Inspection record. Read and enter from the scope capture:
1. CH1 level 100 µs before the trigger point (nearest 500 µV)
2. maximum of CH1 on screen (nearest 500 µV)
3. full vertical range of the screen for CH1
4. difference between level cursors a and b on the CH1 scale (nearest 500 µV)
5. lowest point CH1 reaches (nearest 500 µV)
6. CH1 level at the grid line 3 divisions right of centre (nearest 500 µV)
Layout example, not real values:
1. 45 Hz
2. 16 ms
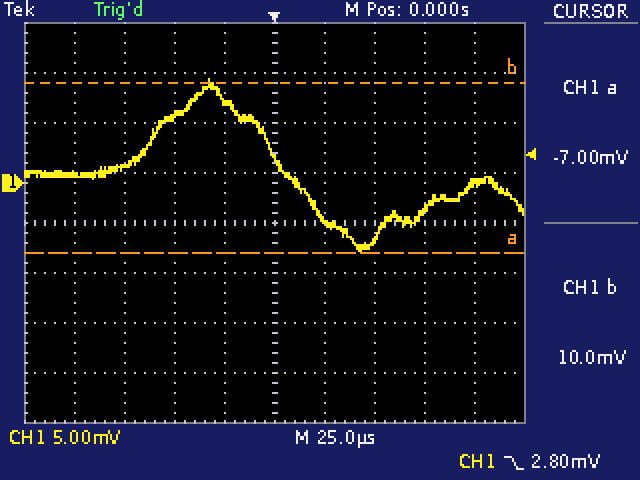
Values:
1. 1.0 mV
2. 10.5 mV
3. 40 mV
4. 17.0 mV
5. -7.0 mV
6. -2.5 mV
